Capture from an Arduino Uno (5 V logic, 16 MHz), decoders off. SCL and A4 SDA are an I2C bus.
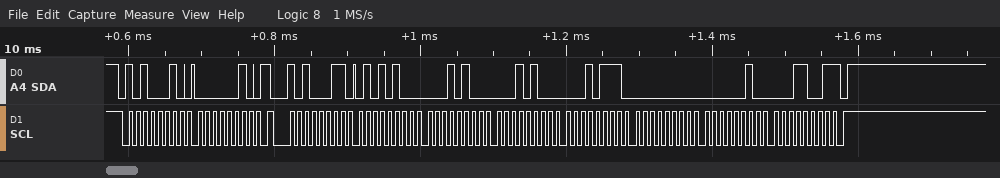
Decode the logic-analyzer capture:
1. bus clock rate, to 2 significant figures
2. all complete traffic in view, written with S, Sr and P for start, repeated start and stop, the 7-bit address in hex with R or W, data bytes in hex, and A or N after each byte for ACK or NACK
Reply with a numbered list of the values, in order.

1. 100 kHz
2. S 51W A 02 A Sr 51R A 54 A 14 A 14 A 17 A 00 A 02 A 19 N P
